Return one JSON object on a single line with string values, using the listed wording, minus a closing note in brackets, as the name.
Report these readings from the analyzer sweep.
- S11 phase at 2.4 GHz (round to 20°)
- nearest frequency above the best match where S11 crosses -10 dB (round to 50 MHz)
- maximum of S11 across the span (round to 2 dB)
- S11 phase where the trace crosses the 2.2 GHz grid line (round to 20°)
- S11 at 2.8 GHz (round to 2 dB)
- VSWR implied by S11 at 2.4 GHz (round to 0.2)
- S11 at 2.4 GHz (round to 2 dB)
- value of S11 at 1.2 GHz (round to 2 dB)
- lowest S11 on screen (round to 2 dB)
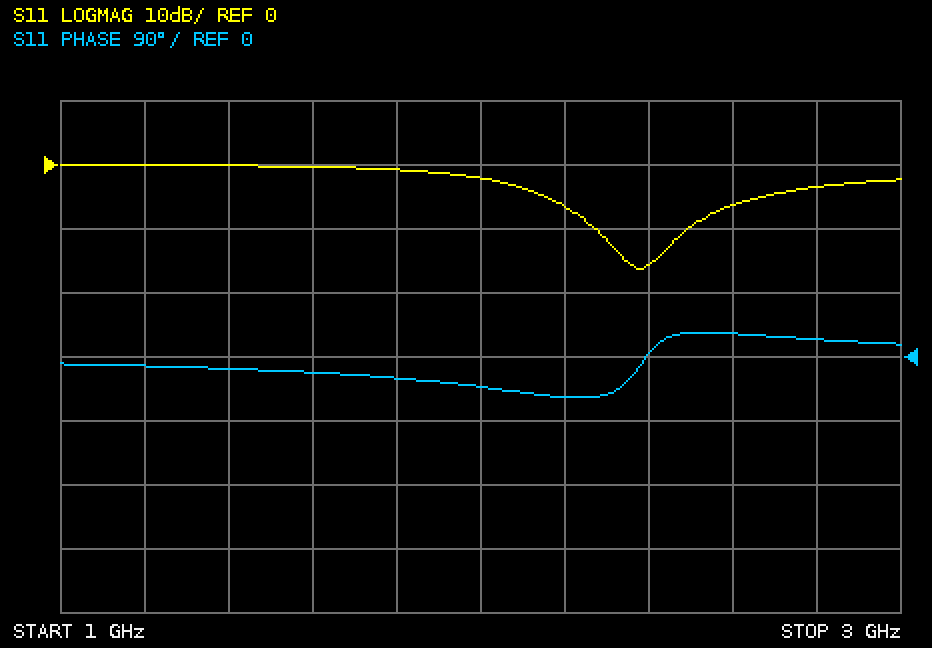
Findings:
{"S11 phase at 2.4 GHz": "0°", "nearest frequency above the best match where S11 crosses -10 dB": "2.50 GHz", "maximum of S11 across the span": "0 dB", "S11 phase where the trace crosses the 2.2 GHz grid line": "-60°", "S11 at 2.8 GHz": "-4 dB", "VSWR implied by S11 at 2.4 GHz": "1.4", "S11 at 2.4 GHz": "-16 dB", "value of S11 at 1.2 GHz": "0 dB", "lowest S11 on screen": "-16 dB"}
